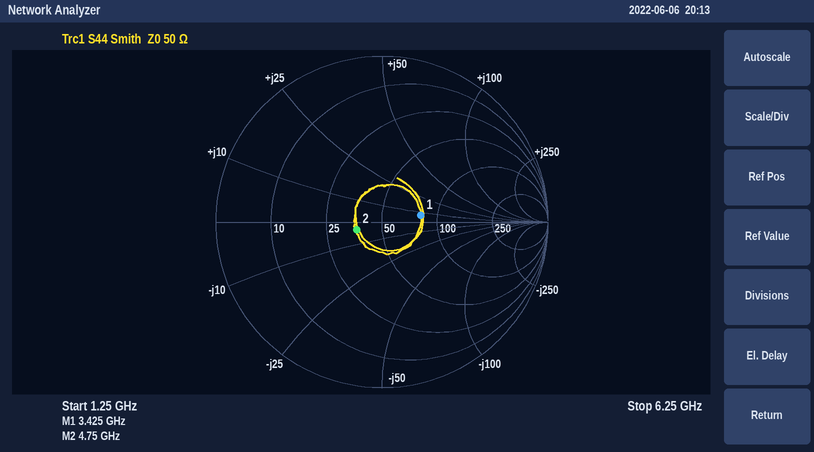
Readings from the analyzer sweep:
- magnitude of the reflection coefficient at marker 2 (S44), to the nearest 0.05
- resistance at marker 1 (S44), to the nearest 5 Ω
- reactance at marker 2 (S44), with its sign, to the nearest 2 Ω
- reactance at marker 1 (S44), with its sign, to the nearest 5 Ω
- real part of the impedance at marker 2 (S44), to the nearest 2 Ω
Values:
0.15
80 Ω
-4 Ω
+5 Ω
36 Ω
